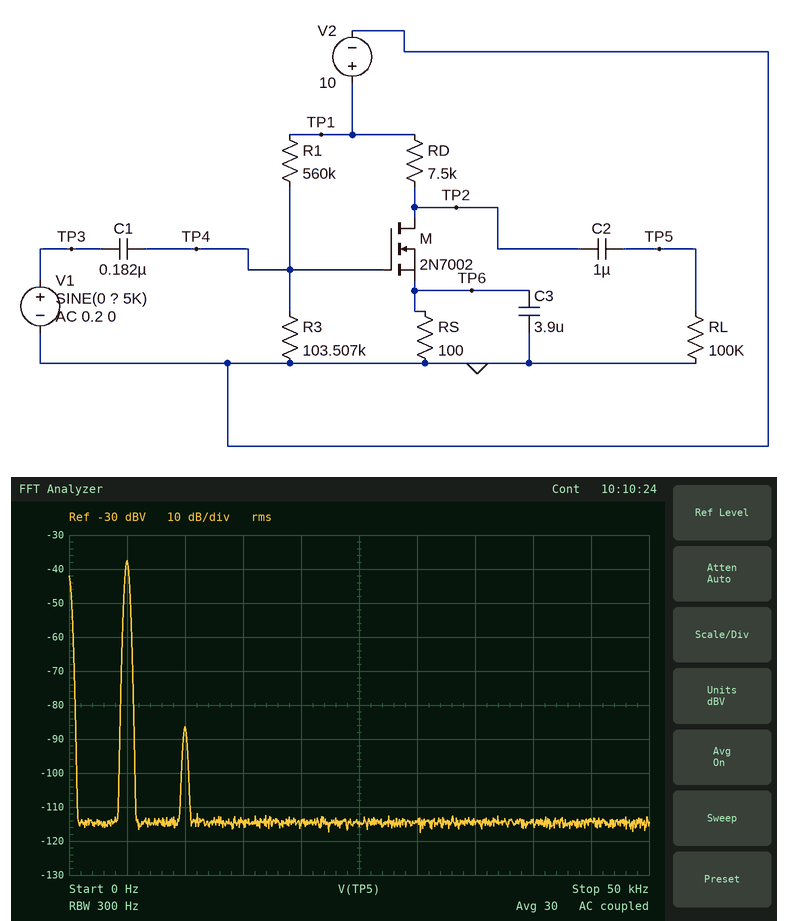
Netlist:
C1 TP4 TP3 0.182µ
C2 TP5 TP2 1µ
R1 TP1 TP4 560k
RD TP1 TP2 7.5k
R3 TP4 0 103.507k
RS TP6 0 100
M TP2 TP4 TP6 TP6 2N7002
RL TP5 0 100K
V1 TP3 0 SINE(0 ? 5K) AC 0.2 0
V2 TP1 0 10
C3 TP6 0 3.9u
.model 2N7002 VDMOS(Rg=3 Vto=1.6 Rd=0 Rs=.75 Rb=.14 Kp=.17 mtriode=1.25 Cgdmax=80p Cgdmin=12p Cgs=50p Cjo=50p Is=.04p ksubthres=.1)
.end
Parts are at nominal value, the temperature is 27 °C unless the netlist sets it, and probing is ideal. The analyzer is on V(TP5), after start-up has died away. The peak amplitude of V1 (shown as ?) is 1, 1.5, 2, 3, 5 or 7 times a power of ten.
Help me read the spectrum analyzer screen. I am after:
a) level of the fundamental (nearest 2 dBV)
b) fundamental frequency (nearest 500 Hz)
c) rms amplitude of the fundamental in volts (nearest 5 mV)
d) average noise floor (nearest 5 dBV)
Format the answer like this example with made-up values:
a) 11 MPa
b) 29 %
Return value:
a) -38 dBV
b) 5.0 kHz
c) 15 mV
d) -115 dBV
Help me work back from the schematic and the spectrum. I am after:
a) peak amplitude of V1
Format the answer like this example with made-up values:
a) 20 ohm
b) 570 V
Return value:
a) 1 mV
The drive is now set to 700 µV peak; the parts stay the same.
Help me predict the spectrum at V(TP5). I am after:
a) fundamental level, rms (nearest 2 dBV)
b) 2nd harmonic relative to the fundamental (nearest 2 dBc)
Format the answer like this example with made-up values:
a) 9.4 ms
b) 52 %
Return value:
a) -40 dBV
b) -52 dBc
